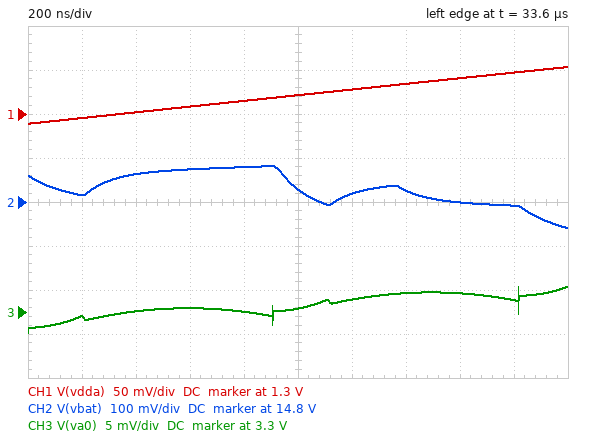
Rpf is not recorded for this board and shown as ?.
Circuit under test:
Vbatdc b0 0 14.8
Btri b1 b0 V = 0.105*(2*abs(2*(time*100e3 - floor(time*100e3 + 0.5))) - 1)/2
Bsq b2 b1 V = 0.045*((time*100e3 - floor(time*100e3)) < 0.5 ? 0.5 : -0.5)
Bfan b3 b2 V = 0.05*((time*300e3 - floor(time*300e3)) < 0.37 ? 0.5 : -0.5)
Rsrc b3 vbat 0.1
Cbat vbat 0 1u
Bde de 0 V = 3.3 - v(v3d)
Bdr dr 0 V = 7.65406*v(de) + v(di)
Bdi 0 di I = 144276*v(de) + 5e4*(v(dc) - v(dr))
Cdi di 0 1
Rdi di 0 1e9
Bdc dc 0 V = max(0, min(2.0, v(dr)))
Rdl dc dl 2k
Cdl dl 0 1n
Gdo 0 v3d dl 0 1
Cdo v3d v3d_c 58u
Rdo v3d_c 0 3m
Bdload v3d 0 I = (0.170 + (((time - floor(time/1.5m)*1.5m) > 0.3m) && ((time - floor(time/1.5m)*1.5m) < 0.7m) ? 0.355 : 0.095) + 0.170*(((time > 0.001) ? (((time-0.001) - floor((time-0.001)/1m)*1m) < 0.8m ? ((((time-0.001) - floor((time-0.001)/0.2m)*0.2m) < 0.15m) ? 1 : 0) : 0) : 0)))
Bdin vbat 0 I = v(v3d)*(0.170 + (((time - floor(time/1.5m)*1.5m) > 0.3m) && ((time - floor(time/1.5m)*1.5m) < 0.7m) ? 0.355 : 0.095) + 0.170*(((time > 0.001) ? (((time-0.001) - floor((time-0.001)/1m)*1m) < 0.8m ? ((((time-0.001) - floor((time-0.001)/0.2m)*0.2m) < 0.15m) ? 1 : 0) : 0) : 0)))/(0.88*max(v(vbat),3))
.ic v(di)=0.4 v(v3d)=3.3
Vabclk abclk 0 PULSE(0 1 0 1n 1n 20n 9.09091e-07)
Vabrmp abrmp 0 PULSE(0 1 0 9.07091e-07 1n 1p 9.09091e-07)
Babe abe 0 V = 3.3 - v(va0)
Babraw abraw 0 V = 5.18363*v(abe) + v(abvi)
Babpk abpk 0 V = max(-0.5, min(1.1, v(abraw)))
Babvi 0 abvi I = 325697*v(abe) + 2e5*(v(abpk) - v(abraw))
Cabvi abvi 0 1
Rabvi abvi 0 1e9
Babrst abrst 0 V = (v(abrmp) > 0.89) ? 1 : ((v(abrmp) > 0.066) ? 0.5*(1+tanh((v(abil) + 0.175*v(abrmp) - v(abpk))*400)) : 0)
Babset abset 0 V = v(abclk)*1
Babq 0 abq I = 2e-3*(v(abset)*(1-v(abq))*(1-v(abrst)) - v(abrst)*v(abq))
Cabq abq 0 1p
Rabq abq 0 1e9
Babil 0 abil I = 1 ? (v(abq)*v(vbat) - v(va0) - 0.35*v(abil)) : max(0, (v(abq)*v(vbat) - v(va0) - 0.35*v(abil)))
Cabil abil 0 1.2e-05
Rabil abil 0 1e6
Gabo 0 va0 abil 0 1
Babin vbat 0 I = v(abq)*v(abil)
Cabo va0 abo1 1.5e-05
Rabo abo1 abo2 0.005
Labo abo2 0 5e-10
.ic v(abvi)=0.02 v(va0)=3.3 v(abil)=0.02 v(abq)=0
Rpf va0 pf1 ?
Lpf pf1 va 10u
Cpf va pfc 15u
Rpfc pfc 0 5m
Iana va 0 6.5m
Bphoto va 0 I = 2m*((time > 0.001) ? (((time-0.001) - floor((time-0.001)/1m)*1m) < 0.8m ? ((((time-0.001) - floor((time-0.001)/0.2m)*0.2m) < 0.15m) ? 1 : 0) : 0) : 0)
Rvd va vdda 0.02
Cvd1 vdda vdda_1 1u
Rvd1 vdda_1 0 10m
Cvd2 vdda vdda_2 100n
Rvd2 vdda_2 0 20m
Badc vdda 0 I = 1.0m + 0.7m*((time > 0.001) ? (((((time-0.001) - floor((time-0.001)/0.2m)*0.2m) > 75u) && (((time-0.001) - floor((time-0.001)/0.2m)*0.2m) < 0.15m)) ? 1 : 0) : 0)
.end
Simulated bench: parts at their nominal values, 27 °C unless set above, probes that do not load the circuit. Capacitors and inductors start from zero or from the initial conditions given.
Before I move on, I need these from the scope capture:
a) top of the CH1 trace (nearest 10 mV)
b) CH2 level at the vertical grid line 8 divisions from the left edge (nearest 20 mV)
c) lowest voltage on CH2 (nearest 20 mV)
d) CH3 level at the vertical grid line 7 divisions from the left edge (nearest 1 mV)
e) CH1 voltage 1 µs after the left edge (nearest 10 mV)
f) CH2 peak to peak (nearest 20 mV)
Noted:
1.35 V
14.80 V
14.74 V
3.302 V
1.32 V
140 mV
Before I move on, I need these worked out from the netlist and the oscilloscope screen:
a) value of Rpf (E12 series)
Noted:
3.9 Ω
